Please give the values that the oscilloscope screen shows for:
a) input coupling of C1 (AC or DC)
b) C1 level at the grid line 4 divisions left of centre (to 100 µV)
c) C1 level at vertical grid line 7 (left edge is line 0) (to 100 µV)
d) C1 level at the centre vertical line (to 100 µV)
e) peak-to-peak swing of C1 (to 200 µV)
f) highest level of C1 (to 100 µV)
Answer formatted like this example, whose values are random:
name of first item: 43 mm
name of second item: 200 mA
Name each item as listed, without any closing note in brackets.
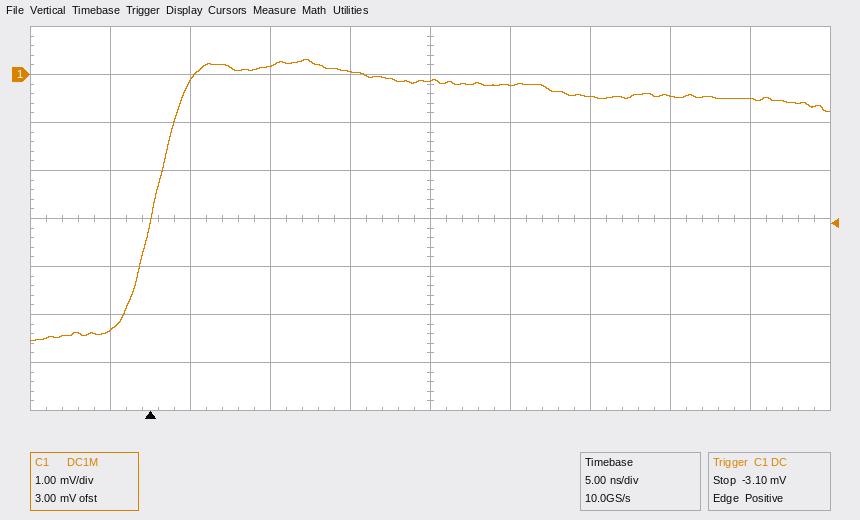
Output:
input coupling of C1: DC
C1 level at the grid line 4 divisions left of centre: -5.3 mV
C1 level at vertical grid line 7 (left edge is line 0): -500 µV
C1 level at the centre vertical line: -100 µV
peak-to-peak swing of C1: 5.8 mV
highest level of C1: 300 µV
